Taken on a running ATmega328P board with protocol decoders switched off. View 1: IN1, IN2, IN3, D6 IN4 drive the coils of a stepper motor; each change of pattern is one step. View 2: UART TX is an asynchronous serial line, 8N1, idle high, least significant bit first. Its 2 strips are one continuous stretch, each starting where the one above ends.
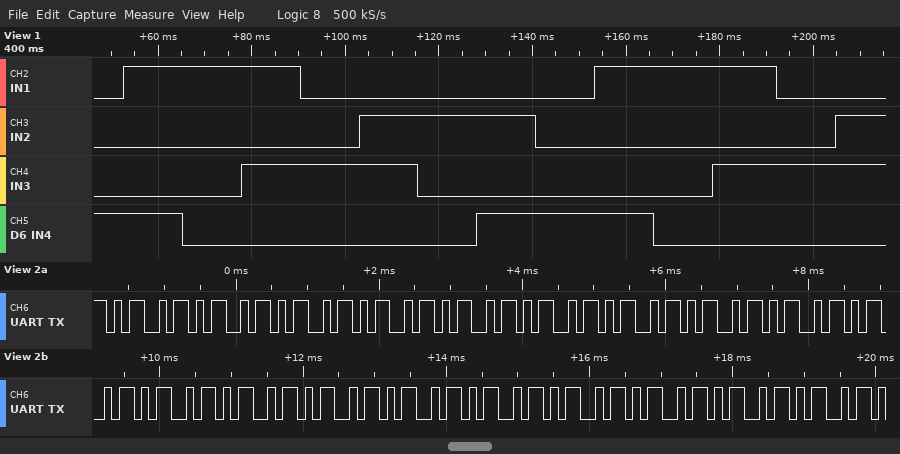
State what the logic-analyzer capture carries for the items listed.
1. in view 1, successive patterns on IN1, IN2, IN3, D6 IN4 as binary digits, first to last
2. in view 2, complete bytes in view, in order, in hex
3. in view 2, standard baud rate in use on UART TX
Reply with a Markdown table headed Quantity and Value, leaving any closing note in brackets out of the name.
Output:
| Quantity | Value |
|---|---|
| in view 1, successive patterns on IN1, IN2, IN3, D6 IN4 as binary digits, first to last | 0001 1001 1000 1010 0010 0110 0100 0101 0001 1001 1000 1010 0010 0110 |
| in view 2, complete bytes in view, in order, in hex | 4D 4D 4D 4D 4D 4D 4D 4D 4D 4D 4D 4D 4D 4D 4D 4D 4D 4D 4D |
| in view 2, standard baud rate in use on UART TX | 9600 baud |
